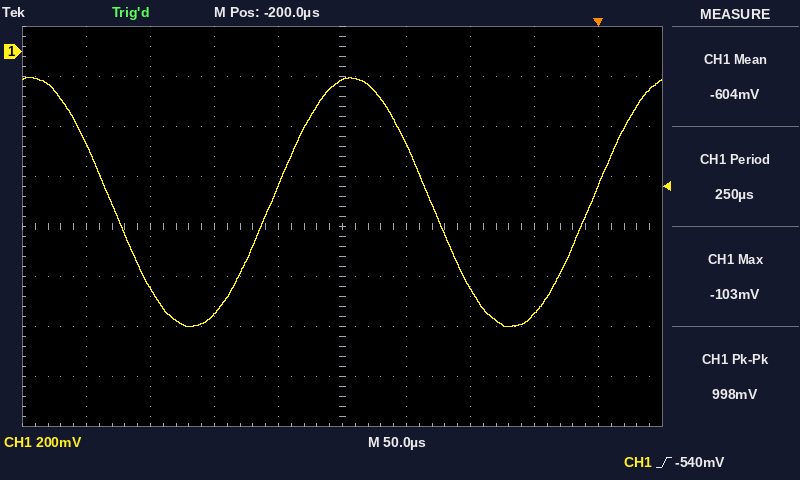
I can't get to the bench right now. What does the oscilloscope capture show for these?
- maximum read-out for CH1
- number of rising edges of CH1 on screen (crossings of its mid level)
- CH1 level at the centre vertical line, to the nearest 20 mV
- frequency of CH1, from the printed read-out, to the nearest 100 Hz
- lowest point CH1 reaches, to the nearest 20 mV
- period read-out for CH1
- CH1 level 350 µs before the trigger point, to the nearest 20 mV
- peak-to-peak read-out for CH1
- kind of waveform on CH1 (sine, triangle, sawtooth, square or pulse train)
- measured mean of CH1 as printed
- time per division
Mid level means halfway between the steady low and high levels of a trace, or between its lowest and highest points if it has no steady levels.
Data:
-103 mV
2
-120 mV
4.0 kHz
-1.10 V
250 µs
-940 mV
998 mV
sine
-604 mV
50 µs
